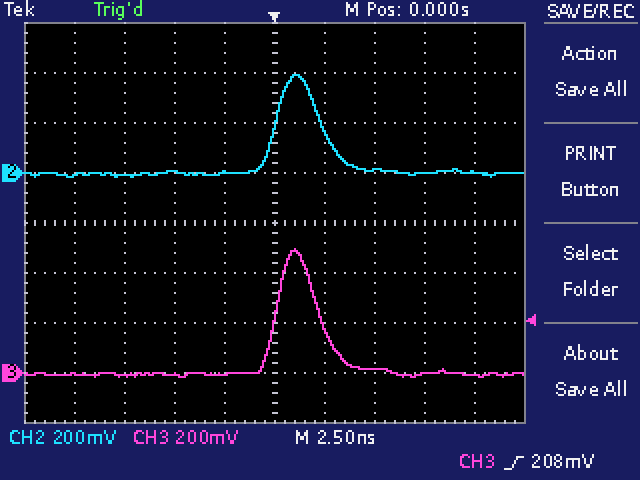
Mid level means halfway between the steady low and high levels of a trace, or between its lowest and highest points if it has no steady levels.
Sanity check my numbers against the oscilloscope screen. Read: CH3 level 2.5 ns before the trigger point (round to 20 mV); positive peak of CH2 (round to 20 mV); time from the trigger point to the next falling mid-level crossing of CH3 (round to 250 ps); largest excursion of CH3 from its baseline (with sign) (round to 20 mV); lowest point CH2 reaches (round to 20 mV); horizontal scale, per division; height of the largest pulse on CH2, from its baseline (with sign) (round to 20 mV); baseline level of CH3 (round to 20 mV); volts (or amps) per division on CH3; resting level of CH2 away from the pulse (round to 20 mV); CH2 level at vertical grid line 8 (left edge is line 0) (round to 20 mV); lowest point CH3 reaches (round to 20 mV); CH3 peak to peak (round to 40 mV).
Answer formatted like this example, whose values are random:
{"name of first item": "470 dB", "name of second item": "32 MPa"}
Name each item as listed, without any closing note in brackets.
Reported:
{"CH3 level 2.5 ns before the trigger point": "0 mV", "positive peak of CH2": "400 mV", "time from the trigger point to the next falling mid-level crossing of CH3": "2.25 ns", "largest excursion of CH3 from its baseline (with sign)": "+500 mV", "lowest point CH2 reaches": "-20 mV", "horizontal scale, per division": "2.5 ns", "height of the largest pulse on CH2, from its baseline (with sign)": "+400 mV", "baseline level of CH3": "0 mV", "volts (or amps) per division on CH3": "200 mV", "resting level of CH2 away from the pulse": "0 mV", "CH2 level at vertical grid line 8 (left edge is line 0)": "0 mV", "lowest point CH3 reaches": "-20 mV", "CH3 peak to peak": "520 mV"}
